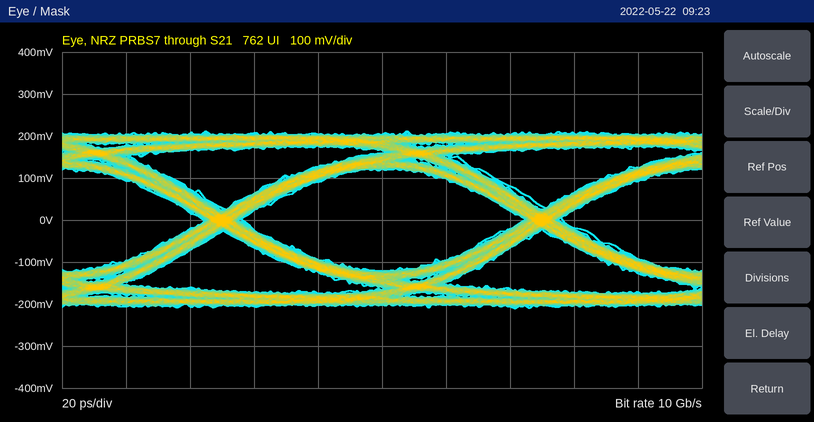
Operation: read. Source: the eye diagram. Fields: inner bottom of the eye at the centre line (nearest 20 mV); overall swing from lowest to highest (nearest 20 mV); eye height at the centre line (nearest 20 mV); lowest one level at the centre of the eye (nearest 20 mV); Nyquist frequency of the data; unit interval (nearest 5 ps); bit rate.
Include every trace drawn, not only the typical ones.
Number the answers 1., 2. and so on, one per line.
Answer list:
1. -120 mV
2. 420 mV
3. 240 mV
4. 120 mV
5. 5 GHz
6. 100 ps
7. 10 Gb/s
